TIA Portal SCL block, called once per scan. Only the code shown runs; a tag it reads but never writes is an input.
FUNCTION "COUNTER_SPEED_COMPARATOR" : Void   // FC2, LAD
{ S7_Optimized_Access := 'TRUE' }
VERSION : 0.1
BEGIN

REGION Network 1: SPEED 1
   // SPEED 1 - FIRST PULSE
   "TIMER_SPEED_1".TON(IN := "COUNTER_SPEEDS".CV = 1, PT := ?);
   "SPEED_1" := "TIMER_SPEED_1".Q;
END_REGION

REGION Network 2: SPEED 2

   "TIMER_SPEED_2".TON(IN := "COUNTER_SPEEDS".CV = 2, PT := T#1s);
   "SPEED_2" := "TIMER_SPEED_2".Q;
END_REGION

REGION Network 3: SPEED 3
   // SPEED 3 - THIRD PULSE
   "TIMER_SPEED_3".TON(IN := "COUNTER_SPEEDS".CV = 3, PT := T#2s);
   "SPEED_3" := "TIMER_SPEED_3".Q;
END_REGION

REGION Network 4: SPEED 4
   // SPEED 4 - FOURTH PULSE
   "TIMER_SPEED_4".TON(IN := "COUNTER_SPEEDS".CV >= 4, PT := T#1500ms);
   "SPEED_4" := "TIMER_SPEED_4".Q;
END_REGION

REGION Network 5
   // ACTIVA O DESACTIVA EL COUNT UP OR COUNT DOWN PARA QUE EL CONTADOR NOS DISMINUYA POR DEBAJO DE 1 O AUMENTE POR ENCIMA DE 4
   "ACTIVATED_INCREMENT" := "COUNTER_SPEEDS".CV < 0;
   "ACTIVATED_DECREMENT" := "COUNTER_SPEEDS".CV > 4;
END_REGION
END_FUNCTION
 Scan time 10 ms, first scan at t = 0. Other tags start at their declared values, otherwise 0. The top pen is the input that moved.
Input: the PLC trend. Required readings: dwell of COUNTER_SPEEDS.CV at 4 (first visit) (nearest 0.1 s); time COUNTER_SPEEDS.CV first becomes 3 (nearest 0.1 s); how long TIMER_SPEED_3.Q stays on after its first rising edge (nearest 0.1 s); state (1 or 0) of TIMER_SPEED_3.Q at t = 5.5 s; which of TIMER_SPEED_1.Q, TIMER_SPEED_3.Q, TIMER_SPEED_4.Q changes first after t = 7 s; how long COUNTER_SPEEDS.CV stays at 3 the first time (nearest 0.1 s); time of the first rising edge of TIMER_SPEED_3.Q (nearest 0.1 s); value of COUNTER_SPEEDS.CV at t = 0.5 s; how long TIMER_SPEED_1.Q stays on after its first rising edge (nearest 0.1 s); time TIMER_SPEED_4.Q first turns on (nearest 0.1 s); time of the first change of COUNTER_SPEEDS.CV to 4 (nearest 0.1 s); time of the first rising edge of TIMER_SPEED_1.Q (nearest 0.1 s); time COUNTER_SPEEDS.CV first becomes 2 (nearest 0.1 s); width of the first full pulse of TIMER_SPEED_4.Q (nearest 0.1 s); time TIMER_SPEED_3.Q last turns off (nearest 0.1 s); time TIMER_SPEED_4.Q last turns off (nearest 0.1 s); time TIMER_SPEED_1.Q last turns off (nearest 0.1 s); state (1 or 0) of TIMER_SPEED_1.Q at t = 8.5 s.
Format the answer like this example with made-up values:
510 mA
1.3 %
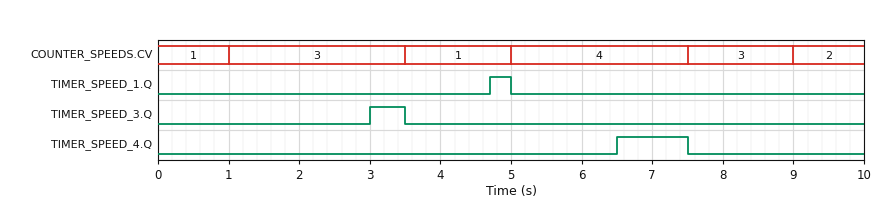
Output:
2.5 s
1.0 s
0.5 s
0
TIMER_SPEED_4.Q
2.5 s
3.0 s
1
0.3 s
6.5 s
5.0 s
4.7 s
9.0 s
1.0 s
3.5 s
7.5 s
5.0 s
0
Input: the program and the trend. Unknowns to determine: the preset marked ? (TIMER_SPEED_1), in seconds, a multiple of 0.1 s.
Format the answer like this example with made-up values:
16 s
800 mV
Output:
1.2 s
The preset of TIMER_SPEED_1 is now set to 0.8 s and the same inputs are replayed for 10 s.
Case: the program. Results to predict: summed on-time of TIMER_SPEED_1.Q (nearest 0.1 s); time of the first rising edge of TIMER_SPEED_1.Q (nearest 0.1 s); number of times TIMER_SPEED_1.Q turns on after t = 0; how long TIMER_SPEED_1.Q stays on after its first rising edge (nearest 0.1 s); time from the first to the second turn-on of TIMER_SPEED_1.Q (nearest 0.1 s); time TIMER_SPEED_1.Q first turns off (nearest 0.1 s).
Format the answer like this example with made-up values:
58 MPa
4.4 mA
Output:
0.9 s
0.8 s
2
0.2 s
3.5 s
1.0 s
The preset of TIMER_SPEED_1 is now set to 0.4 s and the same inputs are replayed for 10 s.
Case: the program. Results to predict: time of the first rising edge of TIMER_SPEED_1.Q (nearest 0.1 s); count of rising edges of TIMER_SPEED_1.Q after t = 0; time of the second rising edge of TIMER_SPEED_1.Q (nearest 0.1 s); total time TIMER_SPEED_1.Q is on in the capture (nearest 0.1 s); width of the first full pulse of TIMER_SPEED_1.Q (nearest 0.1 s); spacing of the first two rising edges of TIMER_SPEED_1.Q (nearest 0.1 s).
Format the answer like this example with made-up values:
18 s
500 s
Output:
0.4 s
2
3.9 s
1.7 s
0.6 s
3.5 s
